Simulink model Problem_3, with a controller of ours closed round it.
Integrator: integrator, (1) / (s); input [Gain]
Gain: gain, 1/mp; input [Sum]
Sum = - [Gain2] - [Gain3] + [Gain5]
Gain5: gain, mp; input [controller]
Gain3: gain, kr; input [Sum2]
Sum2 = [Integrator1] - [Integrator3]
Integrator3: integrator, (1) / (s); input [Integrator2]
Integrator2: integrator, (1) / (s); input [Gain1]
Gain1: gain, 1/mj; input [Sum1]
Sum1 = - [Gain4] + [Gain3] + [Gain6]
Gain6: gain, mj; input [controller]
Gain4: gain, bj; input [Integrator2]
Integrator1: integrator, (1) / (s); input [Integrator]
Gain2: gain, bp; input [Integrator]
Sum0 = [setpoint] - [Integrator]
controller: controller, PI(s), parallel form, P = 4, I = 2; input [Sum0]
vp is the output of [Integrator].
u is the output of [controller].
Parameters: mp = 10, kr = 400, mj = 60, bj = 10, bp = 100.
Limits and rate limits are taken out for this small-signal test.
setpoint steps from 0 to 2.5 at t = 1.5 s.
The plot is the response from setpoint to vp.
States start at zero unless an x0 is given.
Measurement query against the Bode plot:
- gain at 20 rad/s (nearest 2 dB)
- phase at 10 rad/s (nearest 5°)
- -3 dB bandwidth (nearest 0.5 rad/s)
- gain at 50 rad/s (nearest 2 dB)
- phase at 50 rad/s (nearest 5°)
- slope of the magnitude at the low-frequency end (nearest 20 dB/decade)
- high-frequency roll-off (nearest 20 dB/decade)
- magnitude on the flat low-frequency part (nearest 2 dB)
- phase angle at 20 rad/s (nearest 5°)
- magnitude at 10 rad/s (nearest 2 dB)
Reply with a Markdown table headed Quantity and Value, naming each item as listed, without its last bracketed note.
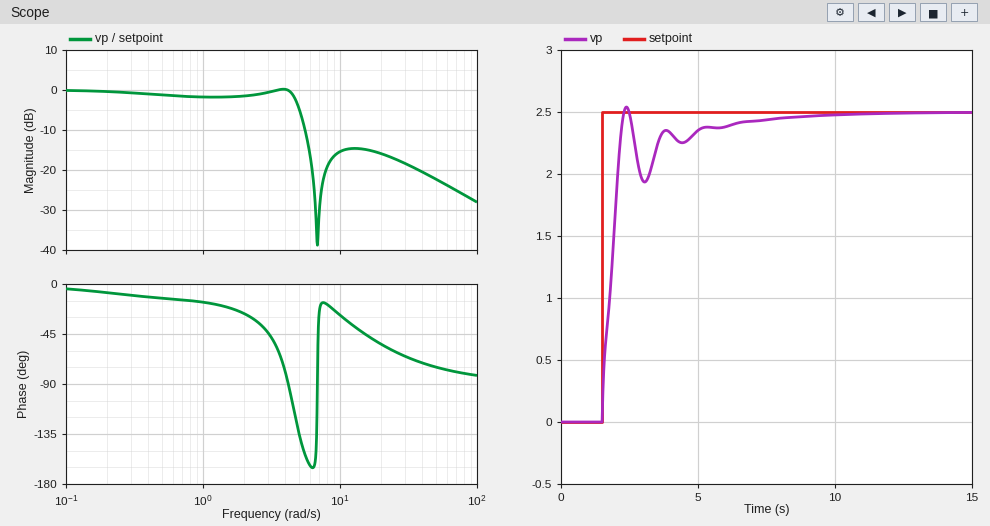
| Quantity | Value |
|---|---|
| gain at 20 rad/s | -16 dB |
| phase at 10 rad/s | -30° |
| -3 dB bandwidth | 5.0 rad/s |
| gain at 50 rad/s | -22 dB |
| phase at 50 rad/s | -75° |
| slope of the magnitude at the low-frequency end | 0 dB/decade |
| high-frequency roll-off | -20 dB/decade |
| magnitude on the flat low-frequency part | 0 dB |
| phase angle at 20 rad/s | -55° |
| magnitude at 10 rad/s | -16 dB |
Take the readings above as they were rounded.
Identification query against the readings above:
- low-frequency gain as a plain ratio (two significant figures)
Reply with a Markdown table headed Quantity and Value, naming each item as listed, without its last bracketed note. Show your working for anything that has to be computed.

| Quantity | Value |
|---|---|
| low-frequency gain as a plain ratio | 10^(0 / 20) = 1.0 |
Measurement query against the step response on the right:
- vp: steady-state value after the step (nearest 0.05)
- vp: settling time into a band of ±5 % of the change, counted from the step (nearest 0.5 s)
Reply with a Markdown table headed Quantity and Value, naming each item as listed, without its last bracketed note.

| Quantity | Value |
|---|---|
| vp: steady-state value after the step | 2.50 |
| vp: settling time into a band of ±5 % of the change, counted from the step | 4.5 s |
